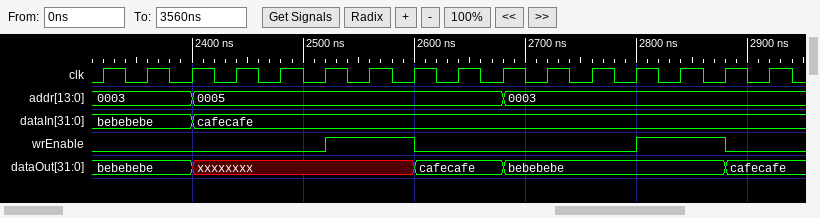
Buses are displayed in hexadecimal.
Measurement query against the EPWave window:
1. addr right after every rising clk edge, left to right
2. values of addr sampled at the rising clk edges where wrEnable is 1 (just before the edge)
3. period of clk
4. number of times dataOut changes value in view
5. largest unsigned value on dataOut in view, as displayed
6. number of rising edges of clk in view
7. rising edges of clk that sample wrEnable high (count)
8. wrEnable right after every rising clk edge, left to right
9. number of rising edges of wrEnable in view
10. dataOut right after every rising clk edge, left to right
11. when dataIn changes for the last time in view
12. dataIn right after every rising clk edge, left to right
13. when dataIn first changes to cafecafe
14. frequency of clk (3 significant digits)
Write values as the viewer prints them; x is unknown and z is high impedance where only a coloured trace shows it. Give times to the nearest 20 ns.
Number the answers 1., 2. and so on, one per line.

1. 0003, 0003, 0005, 0005, 0005, 0005, 0005, 0005, 0005, 0003, 0003, 0003, 0003, 0003, 0003, 0003
2. 0005, 0005, 0003, 0003
3. 40 ns
4. 4
5. cafecafe
6. 16
7. 4
8. 0 0 0 0 0 1 1 0 0 0 0 0 1 1 0 0
9. 2
10. bebebebe, bebebebe, xxxxxxxx, xxxxxxxx, xxxxxxxx, xxxxxxxx, xxxxxxxx, cafecafe, cafecafe, bebebebe, bebebebe, bebebebe, bebebebe, bebebebe, cafecafe, cafecafe
11. 2400 ns
12. bebebebe, bebebebe, cafecafe, cafecafe, cafecafe, cafecafe, cafecafe, cafecafe, cafecafe, cafecafe, cafecafe, cafecafe, cafecafe, cafecafe, cafecafe, cafecafe
13. 2400 ns
14. 25.0 MHz
